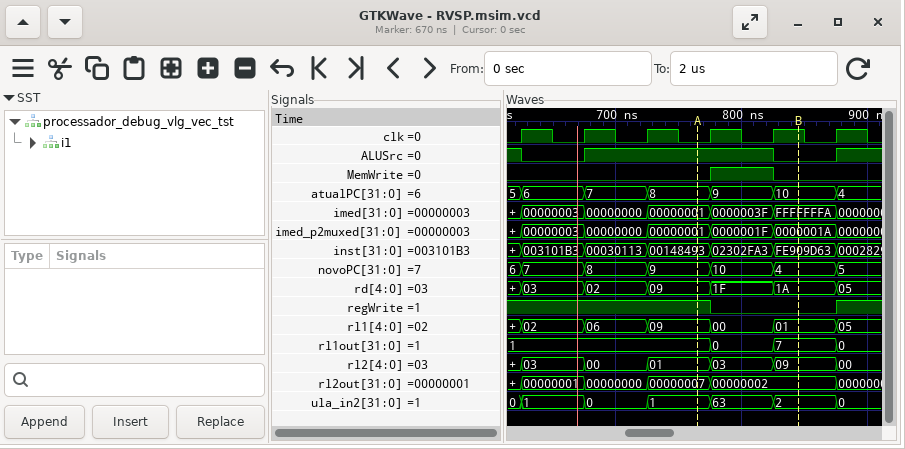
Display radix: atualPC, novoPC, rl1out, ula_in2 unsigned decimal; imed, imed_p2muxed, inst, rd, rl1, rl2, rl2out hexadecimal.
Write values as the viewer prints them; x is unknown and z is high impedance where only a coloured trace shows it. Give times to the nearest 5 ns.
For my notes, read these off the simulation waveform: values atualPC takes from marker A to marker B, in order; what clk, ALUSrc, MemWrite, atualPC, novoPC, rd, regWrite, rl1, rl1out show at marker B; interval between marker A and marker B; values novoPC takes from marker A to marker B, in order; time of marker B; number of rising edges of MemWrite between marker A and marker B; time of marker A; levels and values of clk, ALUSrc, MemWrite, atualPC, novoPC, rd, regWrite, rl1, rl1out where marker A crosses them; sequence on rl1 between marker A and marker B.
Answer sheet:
8, 9, 10
clk=1, ALUSrc=0, MemWrite=0, atualPC=10, novoPC=4, rd=1A, regWrite=0, rl1=01, rl1out=7
80 ns
9, 10, 4
845 ns
1
765 ns
clk=0, ALUSrc=1, MemWrite=0, atualPC=8, novoPC=9, rd=09, regWrite=1, rl1=09, rl1out=1
09, 00, 01
